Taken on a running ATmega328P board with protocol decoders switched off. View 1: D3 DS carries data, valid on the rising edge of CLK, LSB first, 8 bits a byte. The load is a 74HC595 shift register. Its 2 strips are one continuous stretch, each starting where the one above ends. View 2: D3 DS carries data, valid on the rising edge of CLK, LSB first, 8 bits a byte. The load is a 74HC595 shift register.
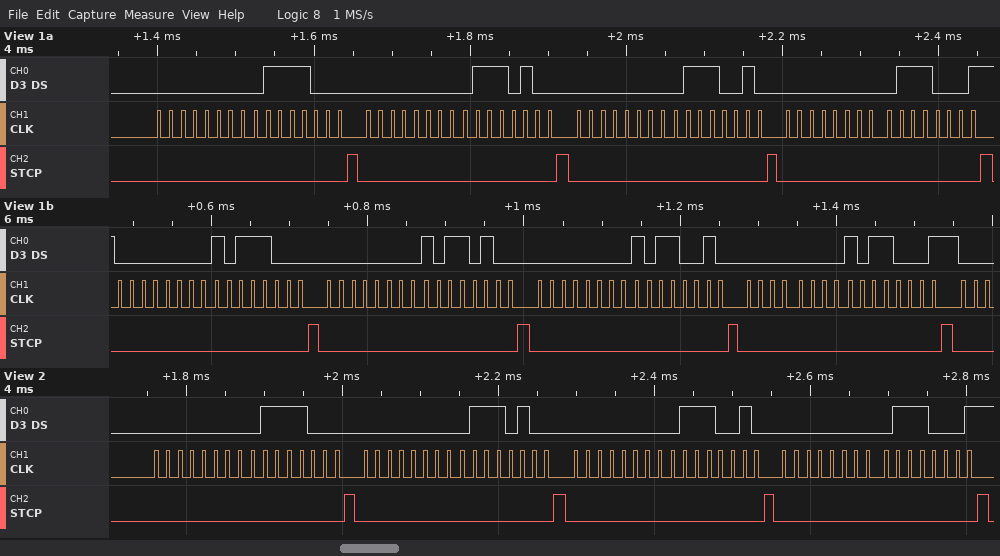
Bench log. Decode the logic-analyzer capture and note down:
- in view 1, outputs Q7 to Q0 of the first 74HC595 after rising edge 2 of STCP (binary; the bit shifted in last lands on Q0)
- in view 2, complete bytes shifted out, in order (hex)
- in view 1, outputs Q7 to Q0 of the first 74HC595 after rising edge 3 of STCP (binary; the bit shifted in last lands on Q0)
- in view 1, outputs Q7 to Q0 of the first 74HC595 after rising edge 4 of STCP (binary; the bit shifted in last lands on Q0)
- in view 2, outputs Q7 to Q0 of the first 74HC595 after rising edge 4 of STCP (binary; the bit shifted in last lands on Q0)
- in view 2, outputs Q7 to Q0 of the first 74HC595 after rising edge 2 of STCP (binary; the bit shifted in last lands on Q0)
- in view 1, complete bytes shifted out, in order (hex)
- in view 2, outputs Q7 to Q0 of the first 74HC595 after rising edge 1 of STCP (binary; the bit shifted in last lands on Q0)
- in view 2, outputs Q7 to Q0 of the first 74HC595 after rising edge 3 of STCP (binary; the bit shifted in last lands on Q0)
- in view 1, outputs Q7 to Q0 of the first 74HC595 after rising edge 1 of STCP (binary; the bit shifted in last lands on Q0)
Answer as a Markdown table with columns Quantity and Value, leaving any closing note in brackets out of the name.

| Quantity | Value |
|---|---|
| in view 1, outputs Q7 to Q0 of the first 74HC595 after rising edge 2 of STCP | 01110100 |
| in view 2, complete bytes shifted out, in order | 00 1E 00 2E 00 4E 00 8E |
| in view 1, outputs Q7 to Q0 of the first 74HC595 after rising edge 3 of STCP | 01110010 |
| in view 1, outputs Q7 to Q0 of the first 74HC595 after rising edge 4 of STCP | 01110001 |
| in view 2, outputs Q7 to Q0 of the first 74HC595 after rising edge 4 of STCP | 01110001 |
| in view 2, outputs Q7 to Q0 of the first 74HC595 after rising edge 2 of STCP | 01110100 |
| in view 1, complete bytes shifted out, in order | 0x00 0x1E 0x00 0x2E 0x00 0x4E 0x00 0x8E 0x00 0x1D 0x00 0x2D 0x00 0x4D 0x00 0x8D |
| in view 2, outputs Q7 to Q0 of the first 74HC595 after rising edge 1 of STCP | 01111000 |
| in view 2, outputs Q7 to Q0 of the first 74HC595 after rising edge 3 of STCP | 01110010 |
| in view 1, outputs Q7 to Q0 of the first 74HC595 after rising edge 1 of STCP | 01111000 |
